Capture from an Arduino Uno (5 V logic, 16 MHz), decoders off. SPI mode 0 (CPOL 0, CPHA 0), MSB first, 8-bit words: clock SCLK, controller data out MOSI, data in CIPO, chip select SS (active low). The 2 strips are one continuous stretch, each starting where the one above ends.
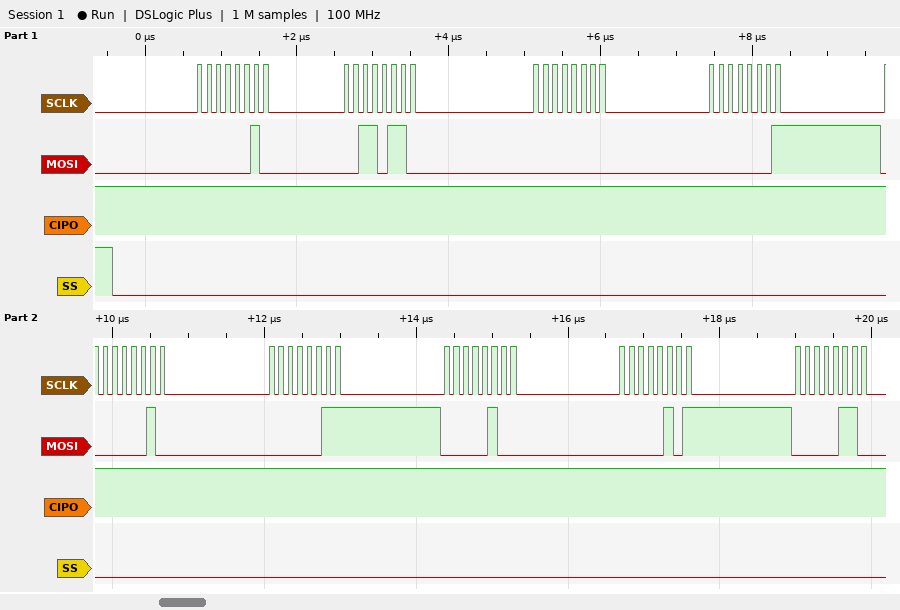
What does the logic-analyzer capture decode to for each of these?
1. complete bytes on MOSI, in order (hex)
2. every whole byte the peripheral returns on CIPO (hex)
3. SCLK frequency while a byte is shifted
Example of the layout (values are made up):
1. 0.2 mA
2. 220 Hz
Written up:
1. 02 36 00 01 02 03 04 05 06
2. FF FF FF FF FF FF FF FF FF
3. 8 MHz
